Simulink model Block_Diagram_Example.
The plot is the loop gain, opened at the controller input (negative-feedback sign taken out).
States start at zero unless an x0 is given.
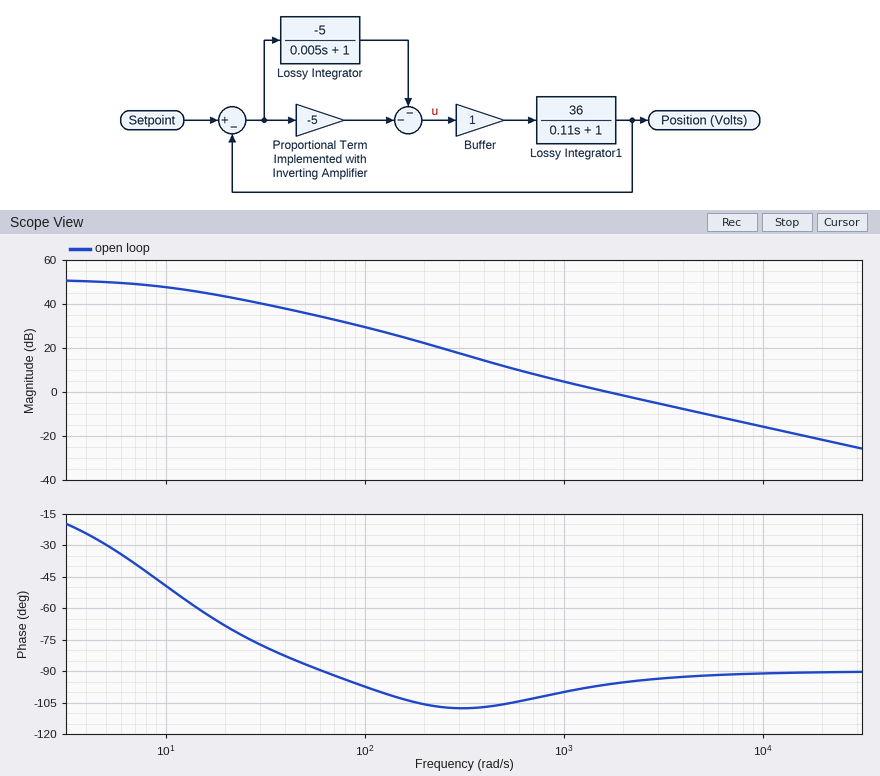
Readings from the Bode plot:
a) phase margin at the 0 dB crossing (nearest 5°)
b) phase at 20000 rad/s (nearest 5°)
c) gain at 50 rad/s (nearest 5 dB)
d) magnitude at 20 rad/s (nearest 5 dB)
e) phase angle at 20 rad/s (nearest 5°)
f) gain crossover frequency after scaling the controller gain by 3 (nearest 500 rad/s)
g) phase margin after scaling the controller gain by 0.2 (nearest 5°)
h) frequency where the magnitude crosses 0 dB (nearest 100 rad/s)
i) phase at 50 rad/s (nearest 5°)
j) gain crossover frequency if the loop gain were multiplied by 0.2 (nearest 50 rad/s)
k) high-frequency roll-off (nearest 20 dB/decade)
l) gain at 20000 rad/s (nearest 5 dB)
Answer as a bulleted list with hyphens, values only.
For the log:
- 85°
- -90°
- 35 dB
- 45 dB
- -70°
- 5000 rad/s
- 75°
- 1700 rad/s
- -85°
- 400 rad/s
- -20 dB/decade
- -20 dB
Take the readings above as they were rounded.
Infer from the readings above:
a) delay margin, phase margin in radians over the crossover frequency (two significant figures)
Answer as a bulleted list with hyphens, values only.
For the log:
- 0.00087 s
